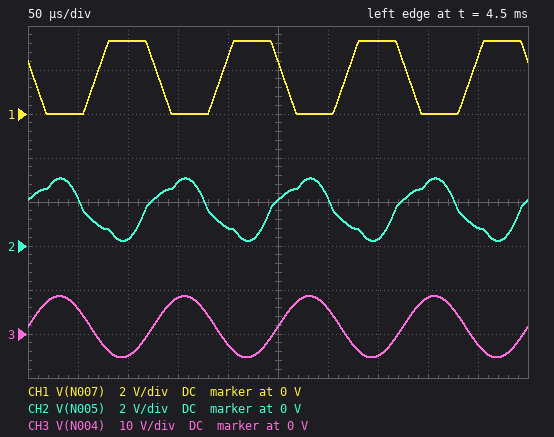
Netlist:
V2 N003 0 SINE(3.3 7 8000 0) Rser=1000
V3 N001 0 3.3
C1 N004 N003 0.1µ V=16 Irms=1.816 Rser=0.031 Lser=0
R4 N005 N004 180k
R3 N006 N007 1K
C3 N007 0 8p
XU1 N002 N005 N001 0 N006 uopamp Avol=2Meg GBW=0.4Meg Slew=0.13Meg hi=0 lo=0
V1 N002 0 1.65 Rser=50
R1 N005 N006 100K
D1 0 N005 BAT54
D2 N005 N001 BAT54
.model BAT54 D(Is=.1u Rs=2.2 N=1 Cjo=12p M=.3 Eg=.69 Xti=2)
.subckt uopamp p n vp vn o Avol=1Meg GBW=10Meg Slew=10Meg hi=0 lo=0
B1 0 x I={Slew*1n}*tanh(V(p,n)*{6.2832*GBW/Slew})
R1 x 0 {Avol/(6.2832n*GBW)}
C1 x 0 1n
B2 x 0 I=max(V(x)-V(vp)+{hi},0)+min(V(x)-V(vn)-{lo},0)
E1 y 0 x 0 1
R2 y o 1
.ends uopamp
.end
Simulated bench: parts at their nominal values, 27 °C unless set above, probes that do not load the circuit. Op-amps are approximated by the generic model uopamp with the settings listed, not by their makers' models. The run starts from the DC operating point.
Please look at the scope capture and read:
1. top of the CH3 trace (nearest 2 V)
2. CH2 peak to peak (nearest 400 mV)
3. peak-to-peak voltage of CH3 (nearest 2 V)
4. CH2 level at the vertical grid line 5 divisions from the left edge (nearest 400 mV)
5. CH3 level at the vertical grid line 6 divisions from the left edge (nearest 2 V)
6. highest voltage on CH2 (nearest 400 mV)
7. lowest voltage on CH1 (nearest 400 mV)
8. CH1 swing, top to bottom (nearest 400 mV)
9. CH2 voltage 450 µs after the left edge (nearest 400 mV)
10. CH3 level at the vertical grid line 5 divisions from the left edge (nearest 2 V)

8 V
2.8 V
14 V
2.0 V
6 V
3.2 V
0 V
3.2 V
800 mV
2 V
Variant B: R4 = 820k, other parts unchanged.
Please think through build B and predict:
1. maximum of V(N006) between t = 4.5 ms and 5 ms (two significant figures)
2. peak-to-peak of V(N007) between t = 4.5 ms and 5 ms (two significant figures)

2.5 V
1.7 V
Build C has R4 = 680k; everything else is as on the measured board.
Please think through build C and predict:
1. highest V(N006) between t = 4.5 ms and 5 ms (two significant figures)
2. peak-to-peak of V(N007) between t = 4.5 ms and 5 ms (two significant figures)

2.7 V
2.1 V
